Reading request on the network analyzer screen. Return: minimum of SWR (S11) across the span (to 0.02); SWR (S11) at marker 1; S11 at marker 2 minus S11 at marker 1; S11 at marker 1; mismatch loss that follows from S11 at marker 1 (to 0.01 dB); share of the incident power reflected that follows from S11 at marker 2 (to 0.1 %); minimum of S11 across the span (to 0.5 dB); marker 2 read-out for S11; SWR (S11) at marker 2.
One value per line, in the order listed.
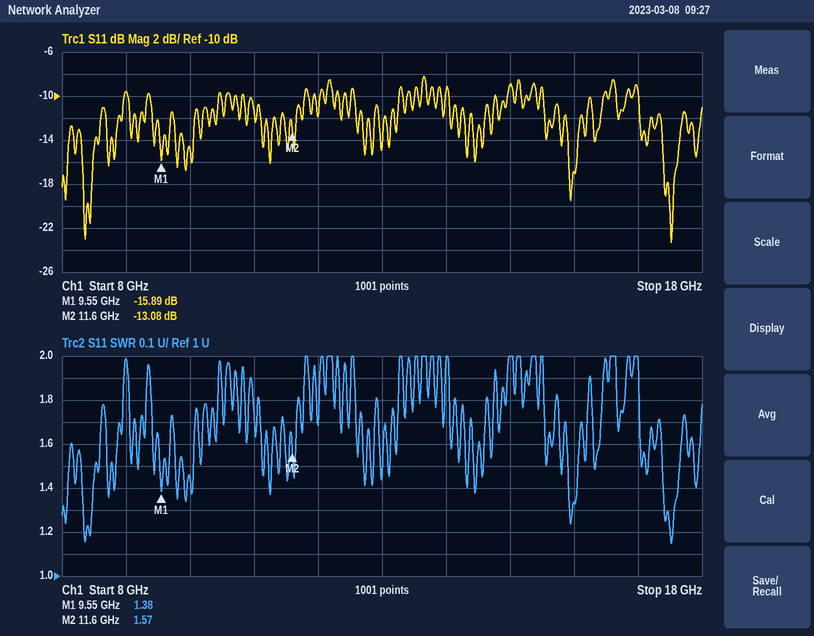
1.14
1.38
2.81 dB
-15.89 dB
0.11 dB
4.9 %
-23.5 dB
-13.08 dB
1.57
